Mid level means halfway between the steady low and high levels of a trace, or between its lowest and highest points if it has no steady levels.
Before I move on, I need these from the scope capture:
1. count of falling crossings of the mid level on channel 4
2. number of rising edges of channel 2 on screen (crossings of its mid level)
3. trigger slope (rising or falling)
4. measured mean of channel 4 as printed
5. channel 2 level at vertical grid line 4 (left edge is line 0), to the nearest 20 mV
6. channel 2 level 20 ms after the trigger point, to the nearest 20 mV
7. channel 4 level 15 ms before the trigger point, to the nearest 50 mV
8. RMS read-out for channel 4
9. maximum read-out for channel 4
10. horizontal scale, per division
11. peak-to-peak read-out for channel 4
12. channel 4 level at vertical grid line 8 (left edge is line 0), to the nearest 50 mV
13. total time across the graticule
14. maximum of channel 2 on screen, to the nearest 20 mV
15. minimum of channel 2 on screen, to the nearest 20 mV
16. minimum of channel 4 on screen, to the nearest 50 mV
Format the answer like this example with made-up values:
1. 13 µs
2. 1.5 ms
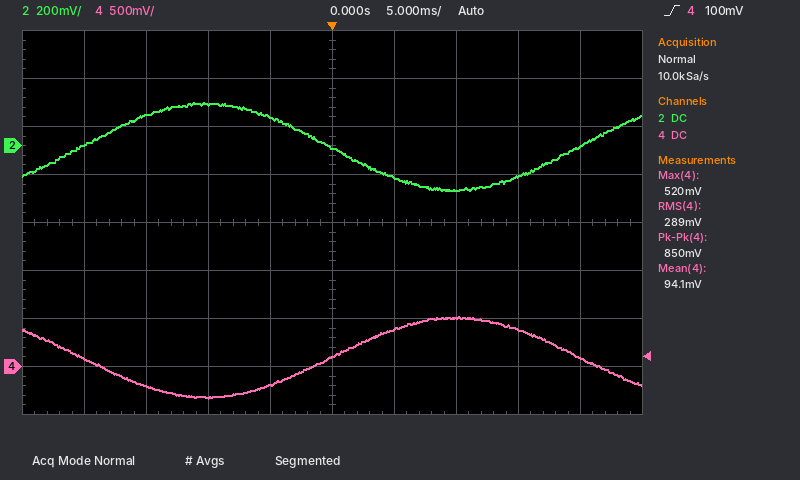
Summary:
1. 2
2. 2
3. rising
4. 94.1 mV
5. 120 mV
6. 0 mV
7. -200 mV
8. 289 mV
9. 520 mV
10. 5 ms
11. 850 mV
12. 400 mV
13. 50 ms
14. 180 mV
15. -180 mV
16. -350 mV
